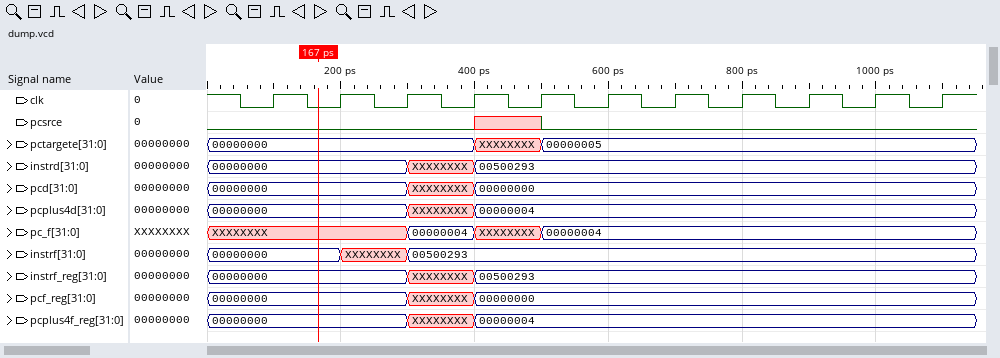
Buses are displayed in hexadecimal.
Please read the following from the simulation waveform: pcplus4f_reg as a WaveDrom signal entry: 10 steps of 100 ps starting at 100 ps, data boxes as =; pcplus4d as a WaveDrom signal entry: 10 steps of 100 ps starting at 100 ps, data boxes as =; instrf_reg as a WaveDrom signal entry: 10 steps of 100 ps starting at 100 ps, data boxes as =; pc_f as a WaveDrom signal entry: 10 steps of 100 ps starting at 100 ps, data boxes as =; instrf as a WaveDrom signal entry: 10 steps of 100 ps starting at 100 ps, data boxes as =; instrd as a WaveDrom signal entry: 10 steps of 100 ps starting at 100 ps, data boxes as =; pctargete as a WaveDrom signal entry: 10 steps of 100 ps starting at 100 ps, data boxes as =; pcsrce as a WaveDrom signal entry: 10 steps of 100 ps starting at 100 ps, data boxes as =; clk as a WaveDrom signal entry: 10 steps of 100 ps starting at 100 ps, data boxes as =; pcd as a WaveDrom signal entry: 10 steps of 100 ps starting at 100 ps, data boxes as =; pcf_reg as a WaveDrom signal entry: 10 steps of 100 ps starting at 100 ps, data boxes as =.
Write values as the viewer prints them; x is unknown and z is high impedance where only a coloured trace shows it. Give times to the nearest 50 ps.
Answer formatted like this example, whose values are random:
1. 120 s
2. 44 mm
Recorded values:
1. {name: 'pcplus4f_reg', wave: '=.x=......', data: '00000000 00000004'}
2. {name: 'pcplus4d', wave: '=.x=......', data: '00000000 00000004'}
3. {name: 'instrf_reg', wave: '=.x=......', data: '00000000 00500293'}
4. {name: 'pc_f', wave: 'x.=x=.....', data: '00000004 00000004'}
5. {name: 'instrf', wave: '=x=.......', data: '00000000 00500293'}
6. {name: 'instrd', wave: '=.x=......', data: '00000000 00500293'}
7. {name: 'pctargete', wave: '=..x=.....', data: '00000000 00000005'}
8. {name: 'pcsrce', wave: '0..x0.....'}
9. {name: 'clk', wave: 'p.........'}
10. {name: 'pcd', wave: '=.x=......', data: '00000000 00000000'}
11. {name: 'pcf_reg', wave: '=.x=......', data: '00000000 00000000'}
